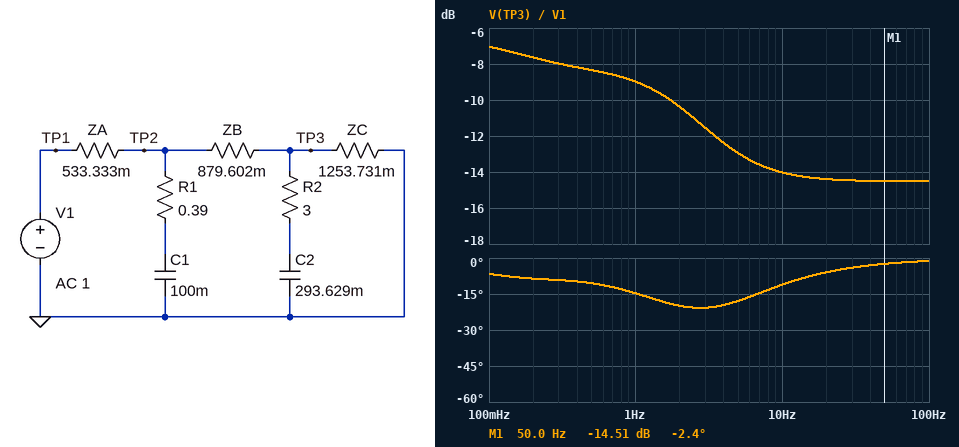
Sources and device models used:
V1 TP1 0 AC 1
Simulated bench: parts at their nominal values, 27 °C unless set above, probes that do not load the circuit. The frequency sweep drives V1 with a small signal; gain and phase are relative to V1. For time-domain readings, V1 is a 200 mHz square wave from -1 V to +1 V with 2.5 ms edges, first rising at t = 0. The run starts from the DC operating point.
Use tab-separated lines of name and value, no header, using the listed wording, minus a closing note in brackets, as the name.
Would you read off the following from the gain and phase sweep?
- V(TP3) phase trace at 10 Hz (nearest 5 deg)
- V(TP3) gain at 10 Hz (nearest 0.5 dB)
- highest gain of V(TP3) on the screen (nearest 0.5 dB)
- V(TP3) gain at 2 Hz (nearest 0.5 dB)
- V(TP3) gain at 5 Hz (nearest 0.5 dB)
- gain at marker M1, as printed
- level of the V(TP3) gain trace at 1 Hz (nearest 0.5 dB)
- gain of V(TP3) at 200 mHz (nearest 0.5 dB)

V(TP3) phase trace at 10 Hz	-10 deg
V(TP3) gain at 10 Hz	-14.0 dB
highest gain of V(TP3) on the screen	-7.0 dB
V(TP3) gain at 2 Hz	-10.5 dB
V(TP3) gain at 5 Hz	-13.0 dB
gain at marker M1, as printed	-14.51 dB
level of the V(TP3) gain trace at 1 Hz	-9.0 dB
gain of V(TP3) at 200 mHz	-7.5 dB
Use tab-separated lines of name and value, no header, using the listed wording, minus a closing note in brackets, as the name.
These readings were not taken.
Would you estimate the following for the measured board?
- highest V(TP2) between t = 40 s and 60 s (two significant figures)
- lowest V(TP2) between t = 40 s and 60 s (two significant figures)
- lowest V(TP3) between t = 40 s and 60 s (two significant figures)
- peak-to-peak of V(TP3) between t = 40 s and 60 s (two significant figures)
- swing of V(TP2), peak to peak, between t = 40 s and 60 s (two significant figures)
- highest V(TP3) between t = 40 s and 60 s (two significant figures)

highest V(TP2) between t = 40 s and 60 s	790 mV
lowest V(TP2) between t = 40 s and 60 s	-790 mV
lowest V(TP3) between t = 40 s and 60 s	-450 mV
peak-to-peak of V(TP3) between t = 40 s and 60 s	910 mV
swing of V(TP2), peak to peak, between t = 40 s and 60 s	1.6 V
highest V(TP3) between t = 40 s and 60 s	450 mV
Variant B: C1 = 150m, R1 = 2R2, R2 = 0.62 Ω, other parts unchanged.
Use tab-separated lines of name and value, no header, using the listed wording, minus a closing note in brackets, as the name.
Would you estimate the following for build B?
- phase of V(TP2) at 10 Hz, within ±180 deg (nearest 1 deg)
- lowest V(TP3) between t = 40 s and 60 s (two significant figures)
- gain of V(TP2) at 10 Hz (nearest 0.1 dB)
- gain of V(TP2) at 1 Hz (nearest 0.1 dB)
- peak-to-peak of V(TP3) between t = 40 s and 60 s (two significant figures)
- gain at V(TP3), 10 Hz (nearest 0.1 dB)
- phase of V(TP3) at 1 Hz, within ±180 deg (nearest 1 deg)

phase of V(TP2) at 10 Hz, within ±180 deg	-1 deg
lowest V(TP3) between t = 40 s and 60 s	-470 mV
gain of V(TP2) at 10 Hz	-4.4 dB
gain of V(TP2) at 1 Hz	-4.0 dB
peak-to-peak of V(TP3) between t = 40 s and 60 s	940 mV
gain at V(TP3), 10 Hz	-14.2 dB
phase of V(TP3) at 1 Hz, within ±180 deg	-21 deg
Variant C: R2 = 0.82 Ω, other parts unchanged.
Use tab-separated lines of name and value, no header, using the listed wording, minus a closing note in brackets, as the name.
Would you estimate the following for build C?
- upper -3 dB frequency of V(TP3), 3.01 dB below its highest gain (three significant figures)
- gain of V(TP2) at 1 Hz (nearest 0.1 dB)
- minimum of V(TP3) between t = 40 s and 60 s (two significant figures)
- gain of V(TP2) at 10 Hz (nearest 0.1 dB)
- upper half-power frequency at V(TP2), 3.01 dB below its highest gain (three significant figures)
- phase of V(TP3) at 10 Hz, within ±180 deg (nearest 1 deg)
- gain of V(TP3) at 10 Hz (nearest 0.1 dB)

upper -3 dB frequency of V(TP3), 3.01 dB below its highest gain	525 mHz
gain of V(TP2) at 1 Hz	-3.5 dB
minimum of V(TP3) between t = 40 s and 60 s	-470 mV
gain of V(TP2) at 10 Hz	-8.3 dB
upper half-power frequency at V(TP2), 3.01 dB below its highest gain	2.10 Hz
phase of V(TP3) at 10 Hz, within ±180 deg	-12 deg
gain of V(TP3) at 10 Hz	-17.2 dB
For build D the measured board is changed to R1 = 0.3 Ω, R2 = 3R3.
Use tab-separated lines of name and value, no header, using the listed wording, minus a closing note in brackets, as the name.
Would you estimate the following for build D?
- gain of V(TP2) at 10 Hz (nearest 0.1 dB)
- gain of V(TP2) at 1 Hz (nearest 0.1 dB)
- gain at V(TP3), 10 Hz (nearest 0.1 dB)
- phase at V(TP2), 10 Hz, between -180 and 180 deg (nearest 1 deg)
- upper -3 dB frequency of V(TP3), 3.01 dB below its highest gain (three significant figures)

gain of V(TP2) at 10 Hz	-8.9 dB
gain of V(TP2) at 1 Hz	-2.9 dB
gain at V(TP3), 10 Hz	-14.8 dB
phase at V(TP2), 10 Hz, between -180 and 180 deg	-15 deg
upper -3 dB frequency of V(TP3), 3.01 dB below its highest gain	1.61 Hz
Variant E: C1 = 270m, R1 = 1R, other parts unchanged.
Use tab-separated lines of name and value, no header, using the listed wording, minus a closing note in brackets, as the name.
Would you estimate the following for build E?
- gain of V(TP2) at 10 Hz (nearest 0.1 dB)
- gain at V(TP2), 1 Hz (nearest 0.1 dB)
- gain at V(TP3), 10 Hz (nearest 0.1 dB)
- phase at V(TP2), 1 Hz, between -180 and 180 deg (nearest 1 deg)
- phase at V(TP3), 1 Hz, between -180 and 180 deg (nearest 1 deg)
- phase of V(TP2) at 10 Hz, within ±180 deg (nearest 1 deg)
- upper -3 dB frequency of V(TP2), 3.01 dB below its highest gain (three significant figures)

gain of V(TP2) at 10 Hz	-5.3 dB
gain at V(TP2), 1 Hz	-4.7 dB
gain at V(TP3), 10 Hz	-11.3 dB
phase at V(TP2), 1 Hz, between -180 and 180 deg	-8 deg
phase at V(TP3), 1 Hz, between -180 and 180 deg	-10 deg
phase of V(TP2) at 10 Hz, within ±180 deg	-1 deg
upper -3 dB frequency of V(TP2), 3.01 dB below its highest gain	1.42 Hz
